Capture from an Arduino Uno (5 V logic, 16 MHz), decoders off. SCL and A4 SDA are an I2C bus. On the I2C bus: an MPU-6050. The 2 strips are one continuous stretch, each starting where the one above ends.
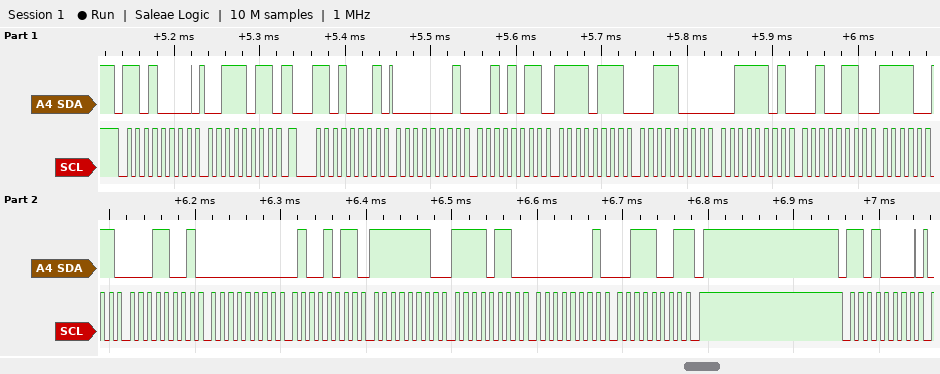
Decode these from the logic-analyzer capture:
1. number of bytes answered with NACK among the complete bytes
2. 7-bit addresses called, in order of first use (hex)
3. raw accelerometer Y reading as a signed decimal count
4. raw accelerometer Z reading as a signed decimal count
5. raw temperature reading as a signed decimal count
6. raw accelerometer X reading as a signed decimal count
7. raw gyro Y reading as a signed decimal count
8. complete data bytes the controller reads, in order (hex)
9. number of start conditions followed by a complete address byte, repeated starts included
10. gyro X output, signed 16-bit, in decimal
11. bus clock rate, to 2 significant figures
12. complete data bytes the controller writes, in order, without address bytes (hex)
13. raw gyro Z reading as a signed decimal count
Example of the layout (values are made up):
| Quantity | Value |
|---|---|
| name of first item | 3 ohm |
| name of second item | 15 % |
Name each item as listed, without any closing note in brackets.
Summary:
| Quantity | Value |
|---|---|
| number of bytes answered with NACK among the complete bytes | 1 |
| 7-bit addresses called, in order of first use | 0x68 |
| raw accelerometer Y reading as a signed decimal count | -2248 |
| raw accelerometer Z reading as a signed decimal count | 15654 |
| raw temperature reading as a signed decimal count | -3303 |
| raw accelerometer X reading as a signed decimal count | 299 |
| raw gyro Y reading as a signed decimal count | -266 |
| complete data bytes the controller reads, in order | 01 2B F7 38 3D 26 F3 19 00 4B FE F6 01 39 |
| number of start conditions followed by a complete address byte, repeated starts included | 3 |
| gyro X output, signed 16-bit, in decimal | 75 |
| bus clock rate, to 2 significant figures | 100 kHz |
| complete data bytes the controller writes, in order, without address bytes | 3B |
| raw gyro Z reading as a signed decimal count | 313 |
